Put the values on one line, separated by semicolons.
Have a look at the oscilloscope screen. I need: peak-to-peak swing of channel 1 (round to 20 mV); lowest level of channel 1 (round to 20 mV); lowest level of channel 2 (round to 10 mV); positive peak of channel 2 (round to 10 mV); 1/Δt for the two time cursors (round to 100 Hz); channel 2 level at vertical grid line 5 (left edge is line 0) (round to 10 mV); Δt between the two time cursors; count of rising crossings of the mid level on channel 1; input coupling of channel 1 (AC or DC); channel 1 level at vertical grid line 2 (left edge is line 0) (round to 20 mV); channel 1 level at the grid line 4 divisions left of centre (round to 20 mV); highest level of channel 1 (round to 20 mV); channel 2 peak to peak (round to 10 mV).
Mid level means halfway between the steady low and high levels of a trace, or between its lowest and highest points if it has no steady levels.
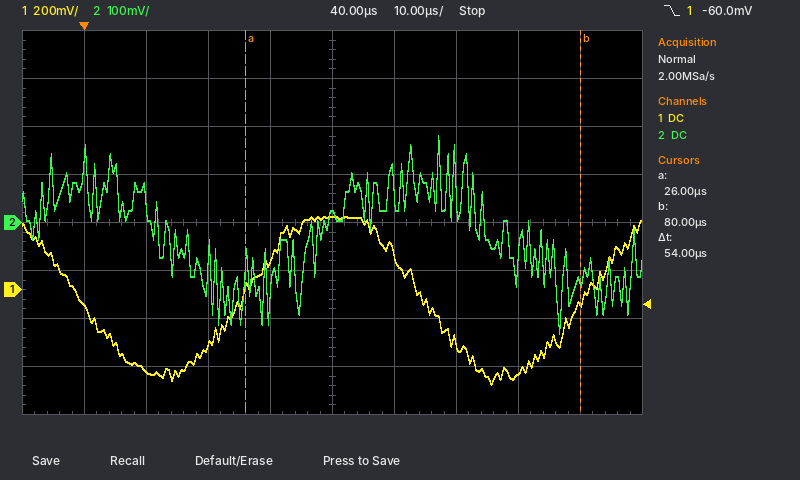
700 mV; -400 mV; -230 mV; 180 mV; 18.5 kHz; 20 mV; 54 µs; 2; DC; -340 mV; -60 mV; 300 mV; 410 mV
